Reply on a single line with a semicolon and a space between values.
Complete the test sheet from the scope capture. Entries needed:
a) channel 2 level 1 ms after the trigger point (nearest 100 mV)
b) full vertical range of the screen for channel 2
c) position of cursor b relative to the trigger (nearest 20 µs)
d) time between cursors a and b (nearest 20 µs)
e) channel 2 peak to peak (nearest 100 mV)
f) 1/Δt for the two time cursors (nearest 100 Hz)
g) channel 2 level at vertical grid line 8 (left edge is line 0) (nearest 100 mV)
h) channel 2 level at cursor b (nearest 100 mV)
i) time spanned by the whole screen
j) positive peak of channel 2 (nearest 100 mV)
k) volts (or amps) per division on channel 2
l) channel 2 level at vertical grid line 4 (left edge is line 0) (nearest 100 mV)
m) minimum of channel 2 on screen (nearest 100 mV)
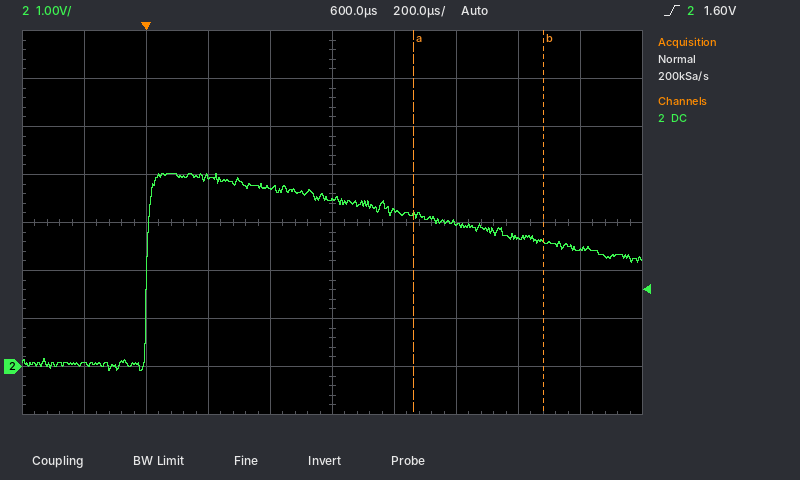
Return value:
3.0 V; 8 V; +1.28 ms; 420 µs; 4.1 V; 2.4 kHz; 2.7 V; 2.6 V; 2 ms; 4.0 V; 1 V; 3.7 V; -100 mV
